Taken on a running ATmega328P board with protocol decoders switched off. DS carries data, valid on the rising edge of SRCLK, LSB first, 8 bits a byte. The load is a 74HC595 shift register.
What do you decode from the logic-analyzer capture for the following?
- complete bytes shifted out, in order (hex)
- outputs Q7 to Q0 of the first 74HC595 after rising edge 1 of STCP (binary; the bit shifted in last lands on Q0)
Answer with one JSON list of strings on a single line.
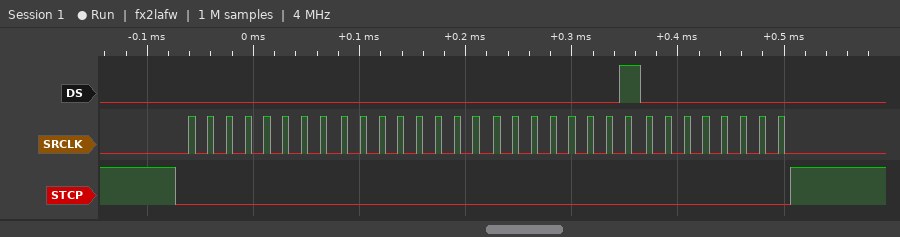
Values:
["00 00 80 00", "00000000"]
